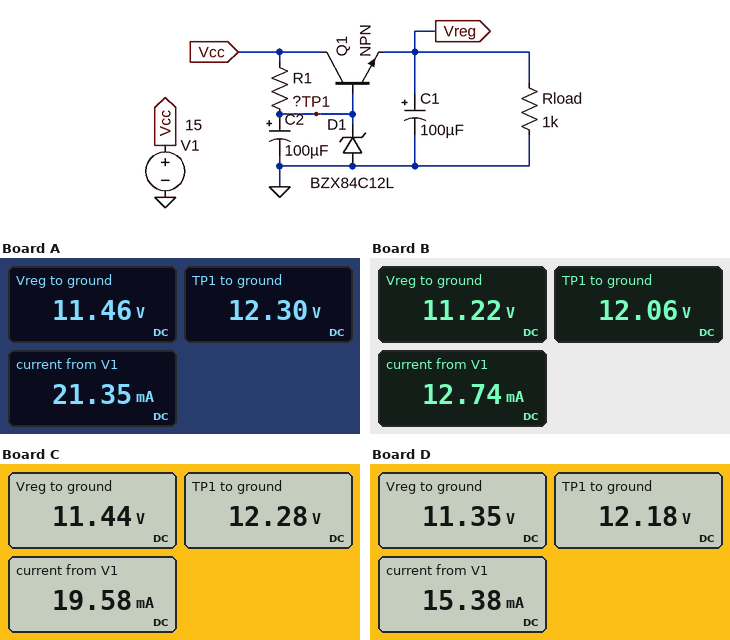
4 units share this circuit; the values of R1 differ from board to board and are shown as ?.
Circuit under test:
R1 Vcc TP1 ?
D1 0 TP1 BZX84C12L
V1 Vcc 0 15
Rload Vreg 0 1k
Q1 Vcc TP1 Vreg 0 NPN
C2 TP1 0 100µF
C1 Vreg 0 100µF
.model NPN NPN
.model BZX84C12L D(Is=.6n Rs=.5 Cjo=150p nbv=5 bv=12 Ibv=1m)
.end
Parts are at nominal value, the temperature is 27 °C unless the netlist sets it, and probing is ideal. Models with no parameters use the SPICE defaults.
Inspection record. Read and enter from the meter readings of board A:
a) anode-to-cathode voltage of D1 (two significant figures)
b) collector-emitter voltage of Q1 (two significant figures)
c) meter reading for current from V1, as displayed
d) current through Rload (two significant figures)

-12 V
3.5 V
21.35 mA
11 mA
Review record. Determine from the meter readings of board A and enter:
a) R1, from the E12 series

270 Ω
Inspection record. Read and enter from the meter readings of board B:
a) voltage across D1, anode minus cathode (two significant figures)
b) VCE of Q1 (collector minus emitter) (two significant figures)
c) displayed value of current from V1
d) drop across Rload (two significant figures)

-12 V
3.8 V
12.74 mA
11 V
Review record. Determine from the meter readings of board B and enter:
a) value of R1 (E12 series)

1.8 kΩ
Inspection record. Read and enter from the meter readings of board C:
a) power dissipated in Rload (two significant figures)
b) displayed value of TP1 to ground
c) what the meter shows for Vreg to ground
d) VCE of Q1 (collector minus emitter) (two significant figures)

130 mW
12.28 V
11.44 V
3.6 V
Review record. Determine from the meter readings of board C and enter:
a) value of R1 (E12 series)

330 Ω
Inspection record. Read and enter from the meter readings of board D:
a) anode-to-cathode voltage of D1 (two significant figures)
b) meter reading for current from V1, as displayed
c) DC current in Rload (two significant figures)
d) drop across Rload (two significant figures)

-12 V
15.38 mA
11 mA
11 V
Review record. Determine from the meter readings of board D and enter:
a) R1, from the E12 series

680 Ω
